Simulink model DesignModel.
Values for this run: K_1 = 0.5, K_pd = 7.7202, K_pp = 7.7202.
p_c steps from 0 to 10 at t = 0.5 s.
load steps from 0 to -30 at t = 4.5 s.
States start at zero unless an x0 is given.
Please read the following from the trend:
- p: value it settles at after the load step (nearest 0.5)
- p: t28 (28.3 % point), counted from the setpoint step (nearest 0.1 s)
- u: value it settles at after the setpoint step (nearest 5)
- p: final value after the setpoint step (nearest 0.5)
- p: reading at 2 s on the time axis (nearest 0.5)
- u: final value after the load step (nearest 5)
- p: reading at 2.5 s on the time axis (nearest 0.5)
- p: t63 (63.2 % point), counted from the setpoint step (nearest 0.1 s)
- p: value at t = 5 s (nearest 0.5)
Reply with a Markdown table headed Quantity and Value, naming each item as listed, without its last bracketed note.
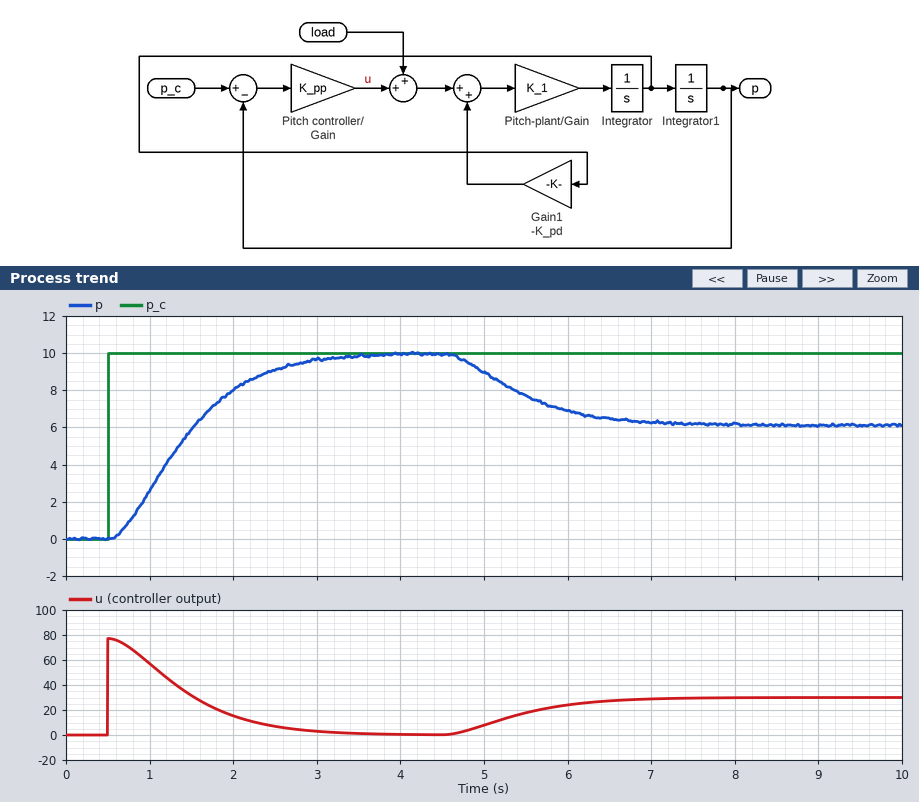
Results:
| Quantity | Value |
|---|---|
| p: value it settles at after the load step | 6.0 |
| p: t28 (28.3 % point), counted from the setpoint step | 0.5 s |
| u: value it settles at after the setpoint step | 0 |
| p: final value after the setpoint step | 10.0 |
| p: reading at 2 s on the time axis | 8.0 |
| u: final value after the load step | 30 |
| p: reading at 2.5 s on the time axis | 9.0 |
| p: t63 (63.2 % point), counted from the setpoint step | 1.1 s |
| p: value at t = 5 s | 9.0 |
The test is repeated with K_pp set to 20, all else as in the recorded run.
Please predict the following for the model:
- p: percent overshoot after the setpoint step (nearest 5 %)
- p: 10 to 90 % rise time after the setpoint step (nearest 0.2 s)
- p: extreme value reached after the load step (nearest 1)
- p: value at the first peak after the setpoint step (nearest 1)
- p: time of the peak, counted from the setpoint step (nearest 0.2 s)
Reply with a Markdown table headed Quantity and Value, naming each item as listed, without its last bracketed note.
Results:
| Quantity | Value |
|---|---|
| p: percent overshoot after the setpoint step | 10 % |
| p: 10 to 90 % rise time after the setpoint step | 0.6 s |
| p: extreme value reached after the load step | 8 |
| p: value at the first peak after the setpoint step | 11 |
| p: time of the peak, counted from the setpoint step | 1.2 s |
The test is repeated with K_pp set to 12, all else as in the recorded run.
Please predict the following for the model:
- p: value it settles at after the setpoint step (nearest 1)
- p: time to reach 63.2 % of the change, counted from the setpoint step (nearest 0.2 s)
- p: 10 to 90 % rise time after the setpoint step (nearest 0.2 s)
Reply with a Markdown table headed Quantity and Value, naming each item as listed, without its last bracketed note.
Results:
| Quantity | Value |
|---|---|
| p: value it settles at after the setpoint step | 10 |
| p: time to reach 63.2 % of the change, counted from the setpoint step | 0.8 s |
| p: 10 to 90 % rise time after the setpoint step | 1.0 s |
